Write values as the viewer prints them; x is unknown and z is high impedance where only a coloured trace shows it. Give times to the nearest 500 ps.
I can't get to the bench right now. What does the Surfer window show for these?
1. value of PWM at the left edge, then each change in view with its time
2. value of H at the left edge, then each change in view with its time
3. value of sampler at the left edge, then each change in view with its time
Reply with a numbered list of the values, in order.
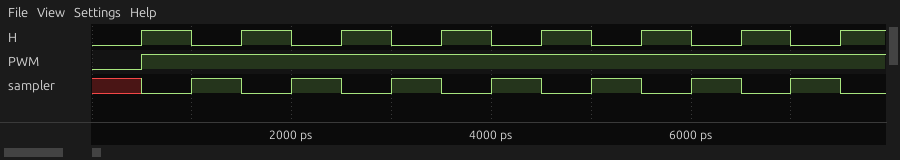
1. 0, 1 at 500 ps
2. 0, 1 at 500 ps, 0 at 1000 ps, 1 at 1500 ps, 0 at 2000 ps, 1 at 2500 ps, 0 at 3000 ps, 1 at 3500 ps, 0 at 4000 ps, 1 at 4500 ps, 0 at 5000 ps, 1 at 5500 ps, 0 at 6000 ps, 1 at 6500 ps, 0 at 7000 ps, 1 at 7500 ps
3. x, 0 at 500 ps, 1 at 1000 ps, 0 at 1500 ps, 1 at 2000 ps, 0 at 2500 ps, 1 at 3000 ps, 0 at 3500 ps, 1 at 4000 ps, 0 at 4500 ps, 1 at 5000 ps, 0 at 5500 ps, 1 at 6000 ps, 0 at 6500 ps, 1 at 7000 ps, 0 at 7500 ps
